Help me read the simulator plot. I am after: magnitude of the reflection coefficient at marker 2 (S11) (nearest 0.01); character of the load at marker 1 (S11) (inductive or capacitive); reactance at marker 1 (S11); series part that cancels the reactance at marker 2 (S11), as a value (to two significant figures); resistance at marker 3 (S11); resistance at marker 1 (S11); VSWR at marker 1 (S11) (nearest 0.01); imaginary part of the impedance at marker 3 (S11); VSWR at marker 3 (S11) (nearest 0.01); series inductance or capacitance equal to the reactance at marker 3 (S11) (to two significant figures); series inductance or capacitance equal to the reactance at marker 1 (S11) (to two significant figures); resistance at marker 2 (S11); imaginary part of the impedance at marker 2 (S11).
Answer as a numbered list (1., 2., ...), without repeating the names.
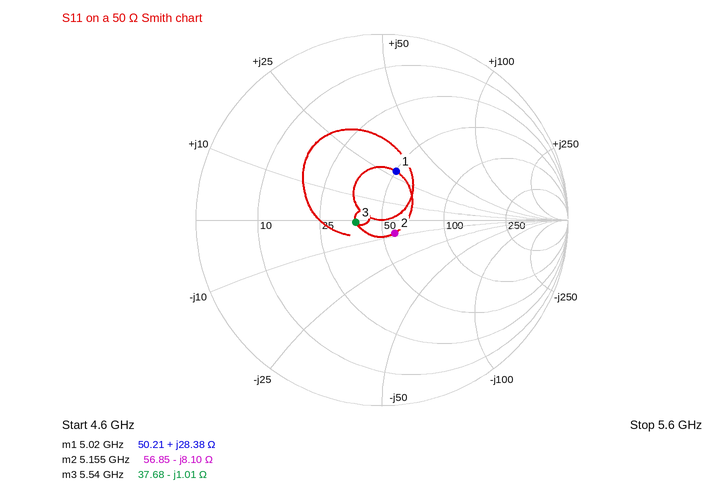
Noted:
1. 0.10
2. inductive
3. +28.38 Ω
4. 250 pH
5. 37.68 Ω
6. 50.21 Ω
7. 1.75
8. -1.01 Ω
9. 1.33
10. 28 pF
11. 900 pH
12. 56.85 Ω
13. -8.10 Ω
